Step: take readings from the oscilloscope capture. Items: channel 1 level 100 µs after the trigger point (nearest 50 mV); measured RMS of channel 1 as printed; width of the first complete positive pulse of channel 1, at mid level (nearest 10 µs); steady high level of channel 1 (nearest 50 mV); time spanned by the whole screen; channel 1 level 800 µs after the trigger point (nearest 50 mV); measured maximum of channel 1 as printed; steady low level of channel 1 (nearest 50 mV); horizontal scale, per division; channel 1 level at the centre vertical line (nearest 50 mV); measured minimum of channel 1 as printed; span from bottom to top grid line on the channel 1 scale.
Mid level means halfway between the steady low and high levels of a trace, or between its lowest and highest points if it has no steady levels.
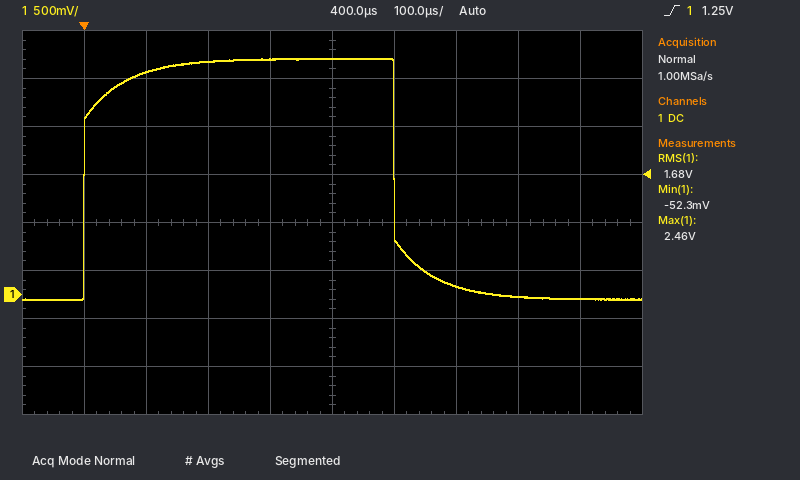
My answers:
2.30 V
1.68 V
500 µs
2.45 V
1 ms
-50 mV
2.46 V
-50 mV
100 µs
2.45 V
-52.3 mV
4 V
